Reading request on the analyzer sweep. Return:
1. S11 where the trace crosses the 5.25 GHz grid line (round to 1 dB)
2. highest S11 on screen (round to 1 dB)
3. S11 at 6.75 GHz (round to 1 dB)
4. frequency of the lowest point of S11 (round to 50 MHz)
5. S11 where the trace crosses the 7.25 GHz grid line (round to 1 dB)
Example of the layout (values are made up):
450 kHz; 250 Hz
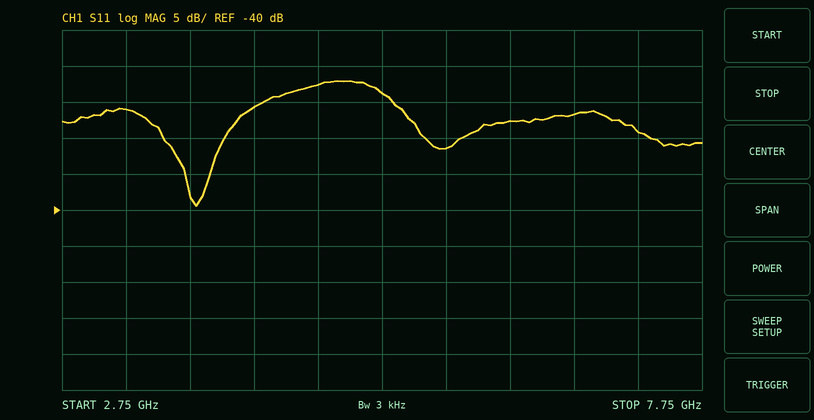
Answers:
-24 dB; -22 dB; -27 dB; 3.80 GHz; -29 dB
